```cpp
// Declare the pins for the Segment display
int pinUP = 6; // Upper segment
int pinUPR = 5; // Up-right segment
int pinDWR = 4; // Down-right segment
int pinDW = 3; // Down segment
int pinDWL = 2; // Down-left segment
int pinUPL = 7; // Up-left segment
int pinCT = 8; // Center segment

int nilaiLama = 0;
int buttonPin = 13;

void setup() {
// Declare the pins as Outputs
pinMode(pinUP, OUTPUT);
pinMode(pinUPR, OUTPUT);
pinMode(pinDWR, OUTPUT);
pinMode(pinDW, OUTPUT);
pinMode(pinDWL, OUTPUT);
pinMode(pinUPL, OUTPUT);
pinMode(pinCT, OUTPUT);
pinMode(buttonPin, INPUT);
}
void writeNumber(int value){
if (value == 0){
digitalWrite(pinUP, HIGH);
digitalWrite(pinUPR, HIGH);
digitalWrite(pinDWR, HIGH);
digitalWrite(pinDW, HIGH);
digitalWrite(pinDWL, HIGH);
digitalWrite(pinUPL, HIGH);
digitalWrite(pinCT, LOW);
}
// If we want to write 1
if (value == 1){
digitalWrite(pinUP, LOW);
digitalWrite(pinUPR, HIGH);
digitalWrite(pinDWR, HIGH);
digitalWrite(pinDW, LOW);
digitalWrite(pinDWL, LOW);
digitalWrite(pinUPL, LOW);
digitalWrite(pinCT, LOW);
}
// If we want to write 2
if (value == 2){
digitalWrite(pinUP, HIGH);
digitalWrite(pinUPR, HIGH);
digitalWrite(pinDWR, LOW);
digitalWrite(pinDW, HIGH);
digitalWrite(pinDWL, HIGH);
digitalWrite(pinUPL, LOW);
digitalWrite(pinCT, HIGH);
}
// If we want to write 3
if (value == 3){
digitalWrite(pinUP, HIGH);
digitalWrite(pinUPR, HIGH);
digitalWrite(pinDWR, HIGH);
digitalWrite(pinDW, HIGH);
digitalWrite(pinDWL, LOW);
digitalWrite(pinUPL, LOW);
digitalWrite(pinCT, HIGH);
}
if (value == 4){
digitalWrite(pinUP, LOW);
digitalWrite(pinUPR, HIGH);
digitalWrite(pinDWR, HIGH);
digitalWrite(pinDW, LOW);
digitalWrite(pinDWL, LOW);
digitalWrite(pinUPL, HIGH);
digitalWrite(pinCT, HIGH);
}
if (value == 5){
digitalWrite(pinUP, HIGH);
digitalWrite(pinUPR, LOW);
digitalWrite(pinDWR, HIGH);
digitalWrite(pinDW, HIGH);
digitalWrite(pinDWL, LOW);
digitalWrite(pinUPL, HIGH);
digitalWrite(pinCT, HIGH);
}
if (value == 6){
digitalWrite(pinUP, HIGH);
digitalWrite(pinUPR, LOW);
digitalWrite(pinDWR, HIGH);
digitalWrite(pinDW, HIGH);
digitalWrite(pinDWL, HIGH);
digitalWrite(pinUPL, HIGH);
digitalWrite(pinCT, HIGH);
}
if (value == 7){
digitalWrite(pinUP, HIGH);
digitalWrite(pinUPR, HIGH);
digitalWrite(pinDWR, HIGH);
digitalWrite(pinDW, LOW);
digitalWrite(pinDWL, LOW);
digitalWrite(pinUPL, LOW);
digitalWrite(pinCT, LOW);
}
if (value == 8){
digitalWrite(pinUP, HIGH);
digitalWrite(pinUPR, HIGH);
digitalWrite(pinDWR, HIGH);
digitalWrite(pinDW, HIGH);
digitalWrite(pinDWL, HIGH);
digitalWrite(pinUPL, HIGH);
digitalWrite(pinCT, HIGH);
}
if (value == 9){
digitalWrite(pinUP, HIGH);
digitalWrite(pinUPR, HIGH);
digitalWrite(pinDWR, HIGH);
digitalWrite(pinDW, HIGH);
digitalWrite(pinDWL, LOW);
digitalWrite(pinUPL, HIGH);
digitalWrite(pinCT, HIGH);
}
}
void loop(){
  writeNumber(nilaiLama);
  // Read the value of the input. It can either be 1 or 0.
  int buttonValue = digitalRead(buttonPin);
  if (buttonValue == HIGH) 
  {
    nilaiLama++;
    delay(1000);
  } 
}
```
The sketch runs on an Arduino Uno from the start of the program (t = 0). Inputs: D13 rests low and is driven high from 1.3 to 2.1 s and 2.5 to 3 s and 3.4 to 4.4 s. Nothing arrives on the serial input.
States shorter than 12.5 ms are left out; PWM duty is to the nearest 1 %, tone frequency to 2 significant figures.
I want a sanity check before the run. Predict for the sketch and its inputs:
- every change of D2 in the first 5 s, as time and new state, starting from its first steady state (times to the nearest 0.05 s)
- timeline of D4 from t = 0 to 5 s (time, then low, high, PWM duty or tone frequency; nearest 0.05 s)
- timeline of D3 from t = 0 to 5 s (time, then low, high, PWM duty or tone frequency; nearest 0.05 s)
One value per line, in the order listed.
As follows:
0 s high; 2.3 s low; 3.5 s high; 4.5 s low
0 s high; 3.5 s low; 4.5 s high
0 s high; 2.3 s low; 3.5 s high
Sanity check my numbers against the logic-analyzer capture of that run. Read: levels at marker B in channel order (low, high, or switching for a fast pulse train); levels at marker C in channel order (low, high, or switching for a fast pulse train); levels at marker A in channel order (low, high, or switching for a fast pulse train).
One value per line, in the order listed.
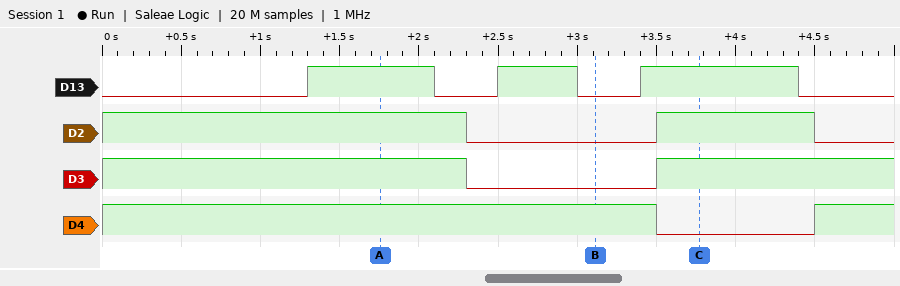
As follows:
D13 low, D2 low, D3 low, D4 high
D13 high, D2 high, D3 high, D4 low
D13 high, D2 high, D3 high, D4 high
